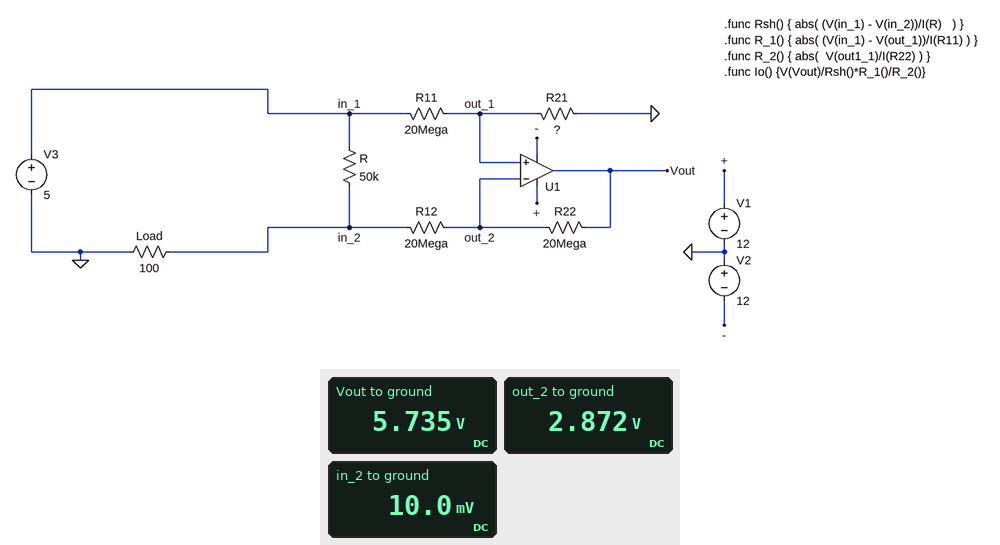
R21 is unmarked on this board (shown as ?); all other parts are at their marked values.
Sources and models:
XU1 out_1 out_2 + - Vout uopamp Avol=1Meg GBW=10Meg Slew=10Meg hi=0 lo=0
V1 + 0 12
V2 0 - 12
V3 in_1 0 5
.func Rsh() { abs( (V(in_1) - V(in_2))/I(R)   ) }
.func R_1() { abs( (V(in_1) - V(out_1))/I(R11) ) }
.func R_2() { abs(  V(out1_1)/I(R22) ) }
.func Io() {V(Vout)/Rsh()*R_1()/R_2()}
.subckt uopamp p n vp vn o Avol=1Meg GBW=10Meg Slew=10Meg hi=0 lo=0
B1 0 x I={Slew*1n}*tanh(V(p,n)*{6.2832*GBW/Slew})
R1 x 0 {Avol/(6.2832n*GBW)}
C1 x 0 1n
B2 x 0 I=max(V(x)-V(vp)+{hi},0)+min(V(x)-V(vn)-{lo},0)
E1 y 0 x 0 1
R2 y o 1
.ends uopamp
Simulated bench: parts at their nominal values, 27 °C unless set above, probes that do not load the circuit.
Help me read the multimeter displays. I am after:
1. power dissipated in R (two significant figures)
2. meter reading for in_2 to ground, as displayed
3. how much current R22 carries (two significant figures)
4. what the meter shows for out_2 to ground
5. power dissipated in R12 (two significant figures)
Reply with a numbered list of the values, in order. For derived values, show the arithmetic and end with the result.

1. (5 V - 10 mV)^2 / 50 kΩ = 500 µW
2. 10.0 mV
3. (5.735 V - 2.872 V) / 20 MΩ = 140 nA
4. 2.872 V
5. (2.872 V - 10 mV)^2 / 20 MΩ = 410 nW
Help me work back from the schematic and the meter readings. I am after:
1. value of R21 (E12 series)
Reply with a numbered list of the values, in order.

1. 27 MΩ
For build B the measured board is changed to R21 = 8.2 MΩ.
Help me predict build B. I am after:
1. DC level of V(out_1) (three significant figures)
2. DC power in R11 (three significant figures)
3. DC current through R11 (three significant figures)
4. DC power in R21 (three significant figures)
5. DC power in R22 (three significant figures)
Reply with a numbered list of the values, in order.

1. 1.45 V
2. 629 nW
3. 177 nA
4. 258 nW
5. 104 nW
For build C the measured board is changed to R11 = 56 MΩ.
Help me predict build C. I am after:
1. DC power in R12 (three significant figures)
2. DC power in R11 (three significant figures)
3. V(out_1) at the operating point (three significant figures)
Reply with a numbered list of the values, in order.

1. 131 nW
2. 203 nW
3. 1.63 V
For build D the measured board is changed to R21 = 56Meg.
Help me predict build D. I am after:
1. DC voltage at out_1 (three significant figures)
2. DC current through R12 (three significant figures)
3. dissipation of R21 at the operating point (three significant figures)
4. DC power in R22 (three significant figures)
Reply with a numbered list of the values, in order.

1. 3.68 V
2. 184 nA
3. 242 nW
4. 675 nW
